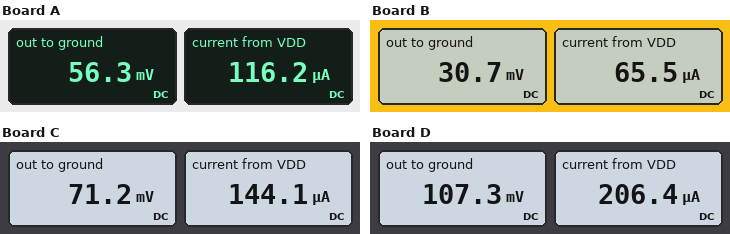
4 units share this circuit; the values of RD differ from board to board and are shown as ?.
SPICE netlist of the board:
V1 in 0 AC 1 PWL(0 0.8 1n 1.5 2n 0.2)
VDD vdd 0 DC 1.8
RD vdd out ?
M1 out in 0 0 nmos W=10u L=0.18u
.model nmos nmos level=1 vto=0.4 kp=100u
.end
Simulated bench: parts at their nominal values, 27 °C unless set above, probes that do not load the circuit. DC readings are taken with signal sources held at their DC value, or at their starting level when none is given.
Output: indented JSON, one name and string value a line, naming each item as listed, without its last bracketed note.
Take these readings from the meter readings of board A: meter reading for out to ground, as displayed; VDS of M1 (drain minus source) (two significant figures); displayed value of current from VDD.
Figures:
{
  "meter reading for out to ground, as displayed": "56.3 mV",
  "VDS of M1 (drain minus source)": "56 mV",
  "displayed value of current from VDD": "116.2 µA"
}
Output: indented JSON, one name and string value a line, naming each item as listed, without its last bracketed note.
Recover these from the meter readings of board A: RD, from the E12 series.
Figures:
{
  "RD, from the E12 series": "15 kΩ"
}
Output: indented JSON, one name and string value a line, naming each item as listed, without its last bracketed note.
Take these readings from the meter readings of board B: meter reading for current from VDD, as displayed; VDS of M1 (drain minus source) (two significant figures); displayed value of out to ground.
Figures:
{
  "meter reading for current from VDD, as displayed": "65.5 µA",
  "VDS of M1 (drain minus source)": "31 mV",
  "displayed value of out to ground": "30.7 mV"
}
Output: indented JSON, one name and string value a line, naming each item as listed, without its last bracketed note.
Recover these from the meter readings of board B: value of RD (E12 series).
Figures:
{
  "value of RD": "27 kΩ"
}
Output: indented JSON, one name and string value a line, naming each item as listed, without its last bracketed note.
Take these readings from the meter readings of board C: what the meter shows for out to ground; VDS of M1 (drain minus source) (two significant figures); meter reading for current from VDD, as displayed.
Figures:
{
  "what the meter shows for out to ground": "71.2 mV",
  "VDS of M1 (drain minus source)": "71 mV",
  "meter reading for current from VDD, as displayed": "144.1 µA"
}
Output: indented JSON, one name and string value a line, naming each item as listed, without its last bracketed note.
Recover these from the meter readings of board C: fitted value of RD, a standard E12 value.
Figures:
{
  "fitted value of RD, a standard E12 value": "12 kΩ"
}
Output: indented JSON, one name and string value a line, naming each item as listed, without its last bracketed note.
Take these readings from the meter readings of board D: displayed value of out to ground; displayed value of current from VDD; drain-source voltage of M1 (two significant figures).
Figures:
{
  "displayed value of out to ground": "107.3 mV",
  "displayed value of current from VDD": "206.4 µA",
  "drain-source voltage of M1": "110 mV"
}
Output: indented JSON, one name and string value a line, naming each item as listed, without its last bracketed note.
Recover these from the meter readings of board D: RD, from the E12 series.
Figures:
{
  "RD, from the E12 series": "8.2 kΩ"
}
